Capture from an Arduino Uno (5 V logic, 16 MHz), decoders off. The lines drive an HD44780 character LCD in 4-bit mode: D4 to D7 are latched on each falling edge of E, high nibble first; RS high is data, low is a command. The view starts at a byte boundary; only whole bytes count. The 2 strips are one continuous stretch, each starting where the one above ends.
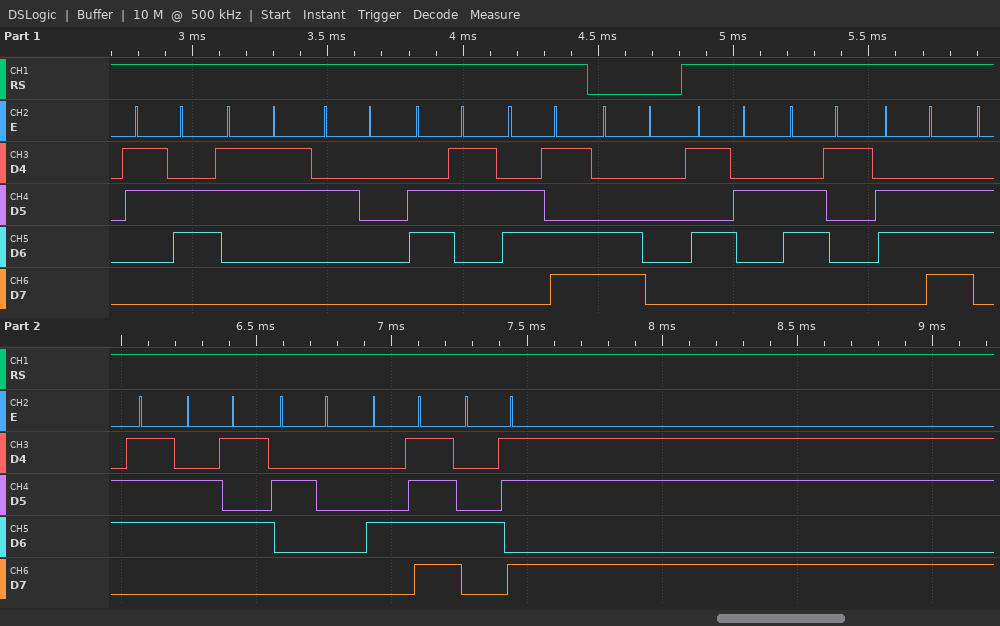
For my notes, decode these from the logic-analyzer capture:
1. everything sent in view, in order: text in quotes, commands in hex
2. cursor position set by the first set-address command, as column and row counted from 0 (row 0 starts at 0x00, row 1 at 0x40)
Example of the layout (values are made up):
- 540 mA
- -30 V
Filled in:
- "63 cm" 0xC0 "Range OK"
- column 0, row 1
